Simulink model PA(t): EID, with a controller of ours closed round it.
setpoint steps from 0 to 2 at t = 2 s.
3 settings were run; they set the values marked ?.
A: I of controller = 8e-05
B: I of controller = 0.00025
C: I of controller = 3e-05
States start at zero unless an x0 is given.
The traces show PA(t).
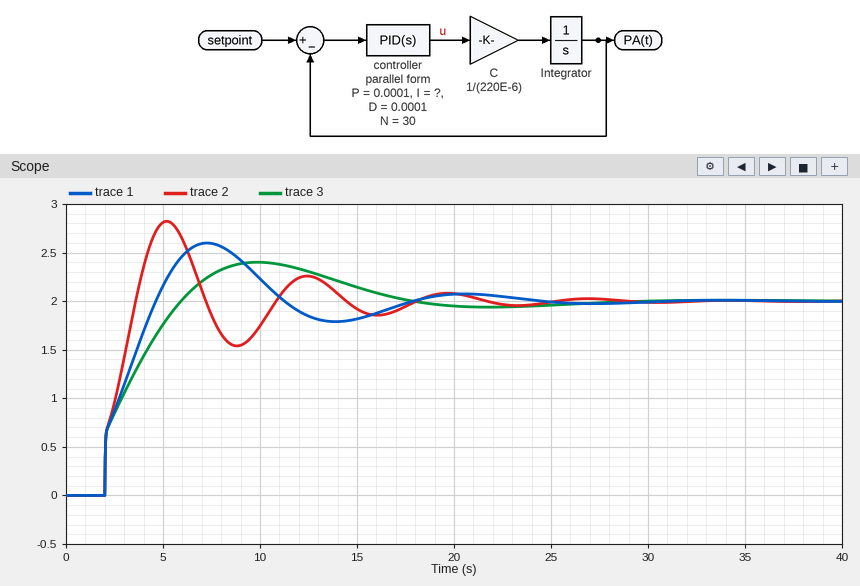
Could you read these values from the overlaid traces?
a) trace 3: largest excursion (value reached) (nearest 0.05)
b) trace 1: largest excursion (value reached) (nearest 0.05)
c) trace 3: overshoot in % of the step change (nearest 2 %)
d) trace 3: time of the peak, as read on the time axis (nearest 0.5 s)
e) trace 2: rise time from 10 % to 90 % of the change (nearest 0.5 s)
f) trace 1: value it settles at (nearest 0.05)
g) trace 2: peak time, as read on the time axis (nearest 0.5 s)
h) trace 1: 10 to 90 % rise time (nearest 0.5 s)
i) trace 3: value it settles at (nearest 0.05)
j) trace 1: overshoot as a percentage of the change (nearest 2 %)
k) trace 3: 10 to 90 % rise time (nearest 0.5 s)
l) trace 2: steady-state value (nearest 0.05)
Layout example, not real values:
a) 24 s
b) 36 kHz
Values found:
a) 2.40
b) 2.60
c) 20 %
d) 10.0 s
e) 1.5 s
f) 2.00
g) 5.0 s
h) 2.0 s
i) 2.00
j) 30 %
k) 3.0 s
l) 2.00
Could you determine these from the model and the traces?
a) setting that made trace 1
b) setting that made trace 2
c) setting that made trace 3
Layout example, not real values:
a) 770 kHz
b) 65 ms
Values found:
a) A
b) B
c) C
